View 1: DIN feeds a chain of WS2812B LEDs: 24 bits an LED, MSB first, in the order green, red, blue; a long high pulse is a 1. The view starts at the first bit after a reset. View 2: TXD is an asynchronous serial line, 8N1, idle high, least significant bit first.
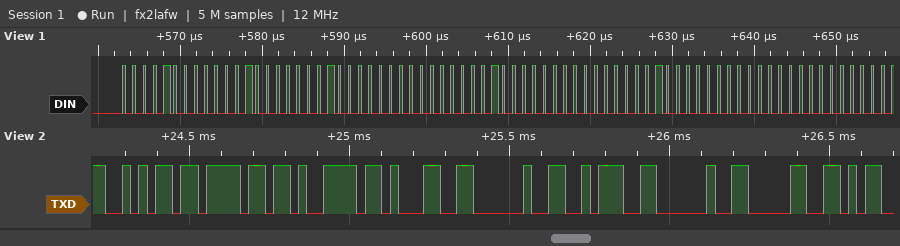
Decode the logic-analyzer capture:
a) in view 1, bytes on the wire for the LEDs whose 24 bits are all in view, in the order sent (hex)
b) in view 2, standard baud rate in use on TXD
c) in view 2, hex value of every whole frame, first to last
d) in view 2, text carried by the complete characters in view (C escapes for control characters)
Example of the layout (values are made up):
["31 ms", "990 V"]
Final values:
["08 08 08 00 08 00 08 00 00", "38400 baud", "6A 6F 79 31 20 3A 20 30", "\"joy1 : 0\""]
